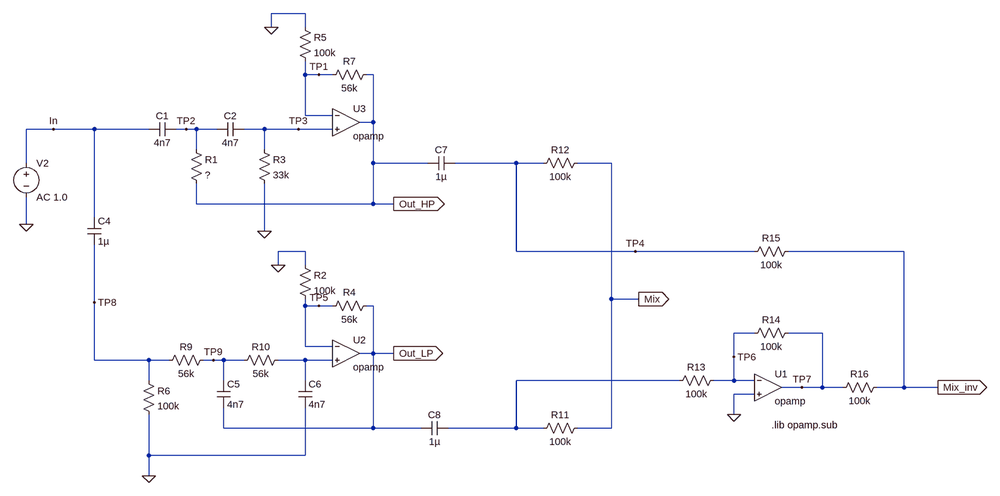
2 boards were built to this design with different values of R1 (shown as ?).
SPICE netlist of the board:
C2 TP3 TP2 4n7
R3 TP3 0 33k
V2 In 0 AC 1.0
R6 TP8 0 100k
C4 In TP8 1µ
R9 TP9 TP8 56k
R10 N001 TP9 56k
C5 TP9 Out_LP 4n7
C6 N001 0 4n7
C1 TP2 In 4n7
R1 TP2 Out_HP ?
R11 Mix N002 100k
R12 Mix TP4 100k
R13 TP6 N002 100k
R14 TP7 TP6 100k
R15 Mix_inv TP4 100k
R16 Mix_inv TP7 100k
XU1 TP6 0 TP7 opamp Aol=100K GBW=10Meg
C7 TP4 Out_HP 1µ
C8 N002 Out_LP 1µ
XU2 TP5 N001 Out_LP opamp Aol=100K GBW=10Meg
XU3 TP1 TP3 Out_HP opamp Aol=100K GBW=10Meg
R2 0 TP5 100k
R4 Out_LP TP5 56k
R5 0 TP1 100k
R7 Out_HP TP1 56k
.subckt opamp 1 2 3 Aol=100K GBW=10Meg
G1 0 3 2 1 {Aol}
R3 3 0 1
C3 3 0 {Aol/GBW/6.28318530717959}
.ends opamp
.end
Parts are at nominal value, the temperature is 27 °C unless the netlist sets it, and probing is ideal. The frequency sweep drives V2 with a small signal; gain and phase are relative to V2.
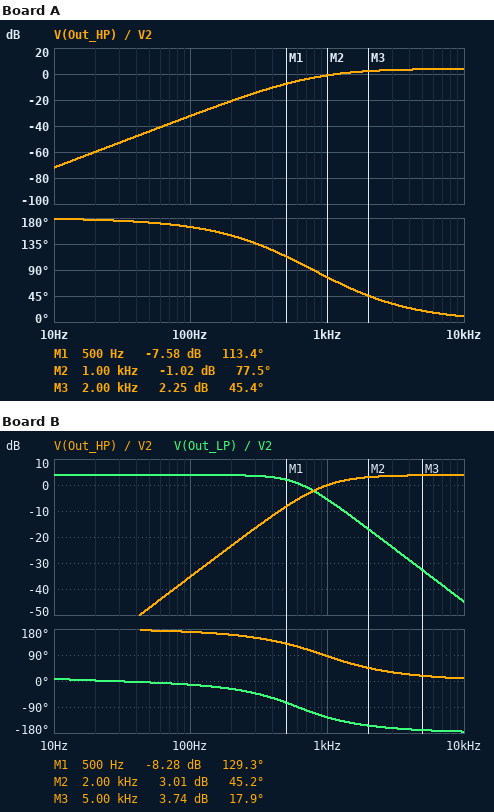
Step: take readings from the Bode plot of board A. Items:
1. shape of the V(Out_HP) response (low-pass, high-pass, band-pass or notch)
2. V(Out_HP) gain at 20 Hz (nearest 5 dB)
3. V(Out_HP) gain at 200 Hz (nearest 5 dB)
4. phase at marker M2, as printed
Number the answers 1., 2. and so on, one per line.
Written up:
1. high-pass
2. -60 dB
3. -20 dB
4. 77.5 deg
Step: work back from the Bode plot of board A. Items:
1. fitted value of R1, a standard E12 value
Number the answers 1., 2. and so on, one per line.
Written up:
1. 56 kΩ
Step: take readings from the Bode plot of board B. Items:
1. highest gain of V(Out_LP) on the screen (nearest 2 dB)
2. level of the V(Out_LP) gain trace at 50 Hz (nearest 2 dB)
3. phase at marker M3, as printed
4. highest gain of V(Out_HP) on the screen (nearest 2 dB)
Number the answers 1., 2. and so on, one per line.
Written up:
1. 4 dB
2. 4 dB
3. 17.9 deg
4. 4 dB
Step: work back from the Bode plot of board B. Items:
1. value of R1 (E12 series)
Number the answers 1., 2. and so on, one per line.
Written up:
1. 39 kΩ
